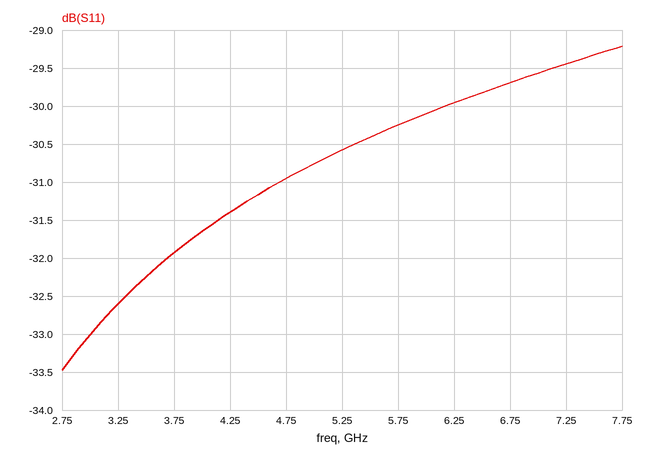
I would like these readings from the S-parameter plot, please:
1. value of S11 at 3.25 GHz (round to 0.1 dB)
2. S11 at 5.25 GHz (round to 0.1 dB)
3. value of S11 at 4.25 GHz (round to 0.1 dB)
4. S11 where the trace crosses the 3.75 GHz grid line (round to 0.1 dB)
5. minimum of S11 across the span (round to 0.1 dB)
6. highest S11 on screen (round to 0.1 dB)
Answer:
-32.6 dB
-30.6 dB
-31.4 dB
-31.9 dB
-33.5 dB
-29.2 dB
